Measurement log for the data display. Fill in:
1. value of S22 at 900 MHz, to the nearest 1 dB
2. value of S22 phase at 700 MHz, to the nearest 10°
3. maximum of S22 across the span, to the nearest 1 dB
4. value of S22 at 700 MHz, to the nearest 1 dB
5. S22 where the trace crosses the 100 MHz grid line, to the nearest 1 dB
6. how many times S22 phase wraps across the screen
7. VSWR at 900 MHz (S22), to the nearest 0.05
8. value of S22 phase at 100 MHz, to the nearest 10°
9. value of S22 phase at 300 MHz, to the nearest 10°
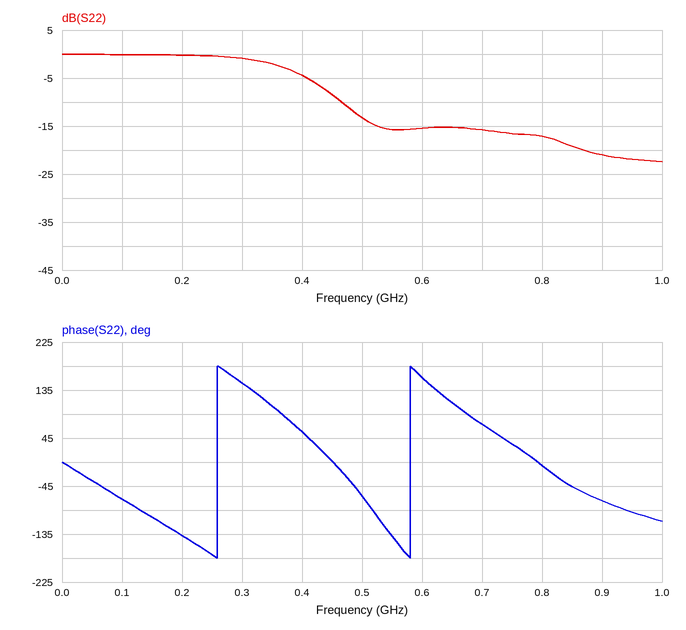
-21 dB
70°
0 dB
-16 dB
0 dB
2
1.20
-70°
150°
